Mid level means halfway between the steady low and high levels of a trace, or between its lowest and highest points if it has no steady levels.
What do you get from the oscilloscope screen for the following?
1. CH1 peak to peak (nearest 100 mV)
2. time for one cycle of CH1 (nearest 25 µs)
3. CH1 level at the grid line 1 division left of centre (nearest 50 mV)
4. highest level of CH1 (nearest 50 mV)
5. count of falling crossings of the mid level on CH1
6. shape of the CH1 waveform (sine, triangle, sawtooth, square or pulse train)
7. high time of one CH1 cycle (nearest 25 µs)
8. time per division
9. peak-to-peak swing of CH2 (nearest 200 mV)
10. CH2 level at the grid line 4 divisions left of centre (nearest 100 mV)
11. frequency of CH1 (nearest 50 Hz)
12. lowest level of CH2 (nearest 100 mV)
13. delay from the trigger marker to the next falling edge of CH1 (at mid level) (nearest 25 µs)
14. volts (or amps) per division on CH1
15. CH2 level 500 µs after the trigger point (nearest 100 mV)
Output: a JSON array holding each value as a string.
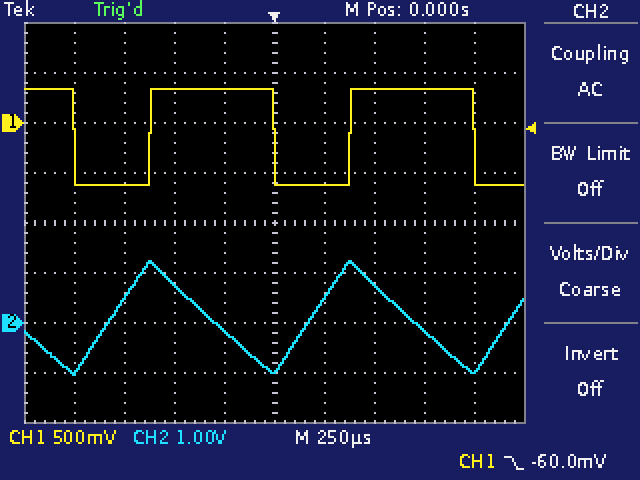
["1.00 V", "1.000 ms", "350 mV", "350 mV", "3", "pulse train", "625 µs", "250 µs", "2.2 V", "-1.0 V", "1.00 kHz", "-1.0 V", "1.000 ms", "500 mV", "800 mV"]
